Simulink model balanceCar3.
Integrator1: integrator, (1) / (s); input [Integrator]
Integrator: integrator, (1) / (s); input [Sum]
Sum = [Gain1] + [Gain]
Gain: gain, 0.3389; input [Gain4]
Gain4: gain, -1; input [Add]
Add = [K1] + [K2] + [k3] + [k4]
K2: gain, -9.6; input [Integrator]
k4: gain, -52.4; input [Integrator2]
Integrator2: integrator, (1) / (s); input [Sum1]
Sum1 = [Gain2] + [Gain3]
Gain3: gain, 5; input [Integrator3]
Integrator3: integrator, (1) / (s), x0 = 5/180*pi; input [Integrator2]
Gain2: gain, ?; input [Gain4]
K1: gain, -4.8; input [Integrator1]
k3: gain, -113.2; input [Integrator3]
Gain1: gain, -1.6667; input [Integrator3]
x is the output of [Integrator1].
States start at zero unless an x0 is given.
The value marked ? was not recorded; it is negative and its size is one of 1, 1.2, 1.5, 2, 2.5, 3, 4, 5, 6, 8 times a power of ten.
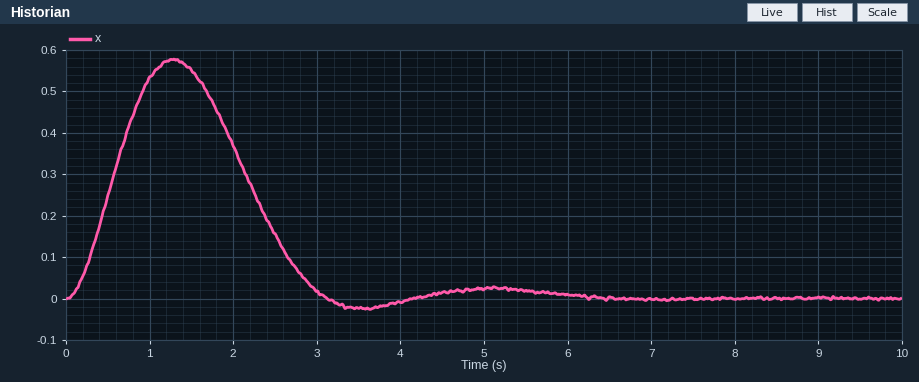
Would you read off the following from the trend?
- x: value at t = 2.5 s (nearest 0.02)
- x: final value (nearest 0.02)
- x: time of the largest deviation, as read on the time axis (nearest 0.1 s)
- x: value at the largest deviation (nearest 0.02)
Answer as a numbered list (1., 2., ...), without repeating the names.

1. 0.16
2. 0.00
3. 1.3 s
4. 0.58
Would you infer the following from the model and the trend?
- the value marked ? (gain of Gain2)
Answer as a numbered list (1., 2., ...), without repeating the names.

1. -0.15
